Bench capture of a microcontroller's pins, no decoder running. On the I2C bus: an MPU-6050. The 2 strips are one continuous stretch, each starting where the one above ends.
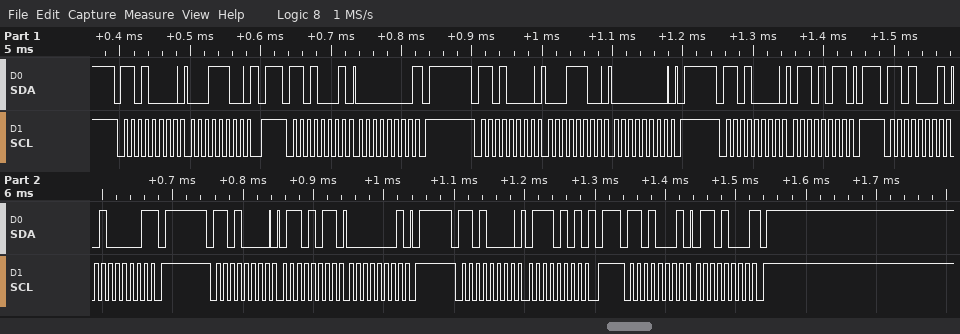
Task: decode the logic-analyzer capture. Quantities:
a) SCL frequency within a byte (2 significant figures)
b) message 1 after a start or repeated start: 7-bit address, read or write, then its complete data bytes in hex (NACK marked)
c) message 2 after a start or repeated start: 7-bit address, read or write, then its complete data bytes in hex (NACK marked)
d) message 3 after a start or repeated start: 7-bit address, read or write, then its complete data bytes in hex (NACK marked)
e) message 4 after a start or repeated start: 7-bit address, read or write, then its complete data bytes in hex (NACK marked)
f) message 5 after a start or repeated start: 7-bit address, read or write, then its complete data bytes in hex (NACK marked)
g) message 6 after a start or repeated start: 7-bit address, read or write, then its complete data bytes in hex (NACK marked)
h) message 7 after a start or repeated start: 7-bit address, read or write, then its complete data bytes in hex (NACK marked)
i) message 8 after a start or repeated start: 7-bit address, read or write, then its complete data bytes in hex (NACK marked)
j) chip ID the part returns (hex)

100 kHz
0x68 write: 1C
0x68 read: 00 NACK
0x68 write: 1C 00
0x68 write: 6B
0x68 read: 41 NACK
0x68 write: 6B 01
0x68 write: 75
0x68 read: 68 NACK
0x68
